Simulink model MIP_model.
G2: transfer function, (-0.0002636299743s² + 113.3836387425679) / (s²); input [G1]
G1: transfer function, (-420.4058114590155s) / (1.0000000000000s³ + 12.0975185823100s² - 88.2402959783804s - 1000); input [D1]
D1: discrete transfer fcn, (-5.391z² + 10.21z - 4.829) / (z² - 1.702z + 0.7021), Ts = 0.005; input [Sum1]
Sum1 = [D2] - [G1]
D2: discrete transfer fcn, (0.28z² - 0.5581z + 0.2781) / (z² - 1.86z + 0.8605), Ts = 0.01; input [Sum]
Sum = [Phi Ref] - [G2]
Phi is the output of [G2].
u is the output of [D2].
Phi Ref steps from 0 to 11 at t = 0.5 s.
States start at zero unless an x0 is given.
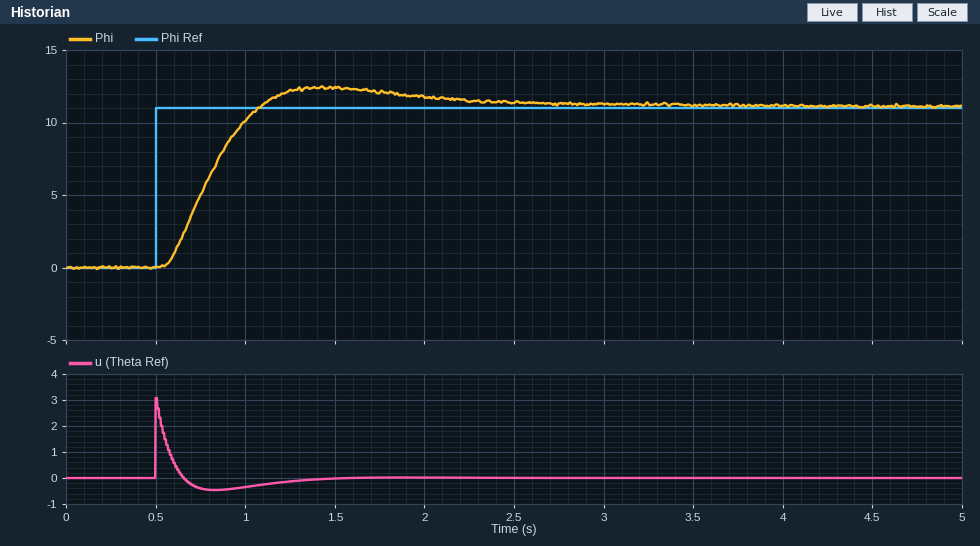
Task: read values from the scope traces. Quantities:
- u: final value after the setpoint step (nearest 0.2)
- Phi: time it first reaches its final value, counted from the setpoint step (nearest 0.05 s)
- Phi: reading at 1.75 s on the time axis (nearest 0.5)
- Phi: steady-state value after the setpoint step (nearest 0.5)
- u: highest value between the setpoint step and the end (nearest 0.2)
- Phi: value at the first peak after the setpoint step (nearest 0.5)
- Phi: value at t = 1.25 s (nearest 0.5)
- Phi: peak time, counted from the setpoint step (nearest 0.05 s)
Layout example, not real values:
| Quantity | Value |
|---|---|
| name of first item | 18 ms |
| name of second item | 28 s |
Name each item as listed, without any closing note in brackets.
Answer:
| Quantity | Value |
|---|---|
| u: final value after the setpoint step | 0.0 |
| Phi: time it first reaches its final value, counted from the setpoint step | 0.60 s |
| Phi: reading at 1.75 s on the time axis | 12.0 |
| Phi: steady-state value after the setpoint step | 11.0 |
| u: highest value between the setpoint step and the end | 3.0 |
| Phi: value at the first peak after the setpoint step | 12.5 |
| Phi: value at t = 1.25 s | 12.0 |
| Phi: peak time, counted from the setpoint step | 0.95 s |
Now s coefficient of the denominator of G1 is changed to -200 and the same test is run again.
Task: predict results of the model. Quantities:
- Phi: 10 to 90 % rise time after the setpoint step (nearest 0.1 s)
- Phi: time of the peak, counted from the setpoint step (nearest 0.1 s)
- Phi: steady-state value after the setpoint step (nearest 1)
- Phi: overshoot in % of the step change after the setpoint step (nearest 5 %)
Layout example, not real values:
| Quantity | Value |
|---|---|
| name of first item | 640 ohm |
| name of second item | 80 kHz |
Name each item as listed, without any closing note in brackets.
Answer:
| Quantity | Value |
|---|---|
| Phi: 10 to 90 % rise time after the setpoint step | 0.3 s |
| Phi: time of the peak, counted from the setpoint step | 0.8 s |
| Phi: steady-state value after the setpoint step | 11 |
| Phi: overshoot in % of the step change after the setpoint step | 10 % |
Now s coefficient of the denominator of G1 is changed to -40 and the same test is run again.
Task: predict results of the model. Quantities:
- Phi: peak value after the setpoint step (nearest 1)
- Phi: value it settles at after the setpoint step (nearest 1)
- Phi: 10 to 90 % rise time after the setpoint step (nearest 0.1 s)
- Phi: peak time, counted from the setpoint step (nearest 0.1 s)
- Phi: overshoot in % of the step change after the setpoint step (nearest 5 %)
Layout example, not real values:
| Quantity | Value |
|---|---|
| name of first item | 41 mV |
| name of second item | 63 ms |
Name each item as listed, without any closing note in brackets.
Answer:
| Quantity | Value |
|---|---|
| Phi: peak value after the setpoint step | 13 |
| Phi: value it settles at after the setpoint step | 11 |
| Phi: 10 to 90 % rise time after the setpoint step | 0.4 s |
| Phi: peak time, counted from the setpoint step | 1.0 s |
| Phi: overshoot in % of the step change after the setpoint step | 15 % |
